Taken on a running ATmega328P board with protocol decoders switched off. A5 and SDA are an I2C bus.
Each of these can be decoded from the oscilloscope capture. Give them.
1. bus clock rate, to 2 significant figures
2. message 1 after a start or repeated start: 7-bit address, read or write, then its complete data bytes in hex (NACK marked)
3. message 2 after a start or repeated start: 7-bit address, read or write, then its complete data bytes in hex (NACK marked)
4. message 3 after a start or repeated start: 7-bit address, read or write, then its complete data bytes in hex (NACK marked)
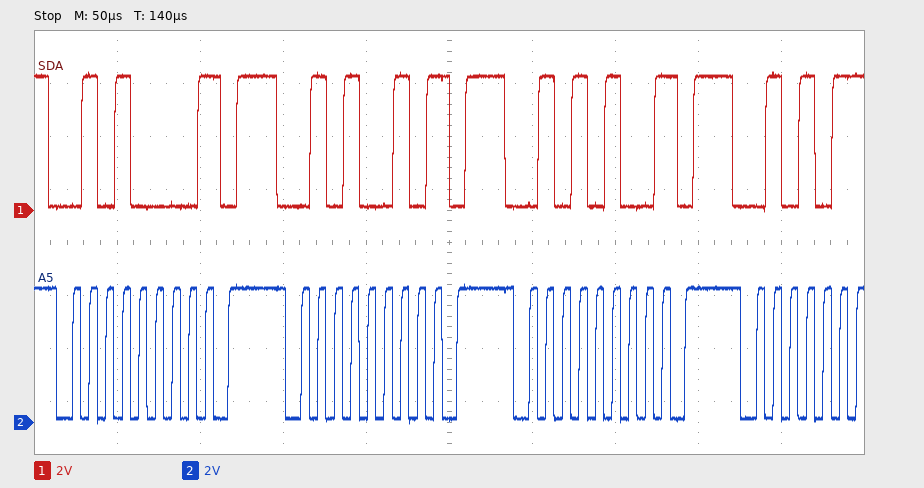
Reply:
100 kHz
0x28 write NACK
0x29 write NACK
0x2A write NACK
